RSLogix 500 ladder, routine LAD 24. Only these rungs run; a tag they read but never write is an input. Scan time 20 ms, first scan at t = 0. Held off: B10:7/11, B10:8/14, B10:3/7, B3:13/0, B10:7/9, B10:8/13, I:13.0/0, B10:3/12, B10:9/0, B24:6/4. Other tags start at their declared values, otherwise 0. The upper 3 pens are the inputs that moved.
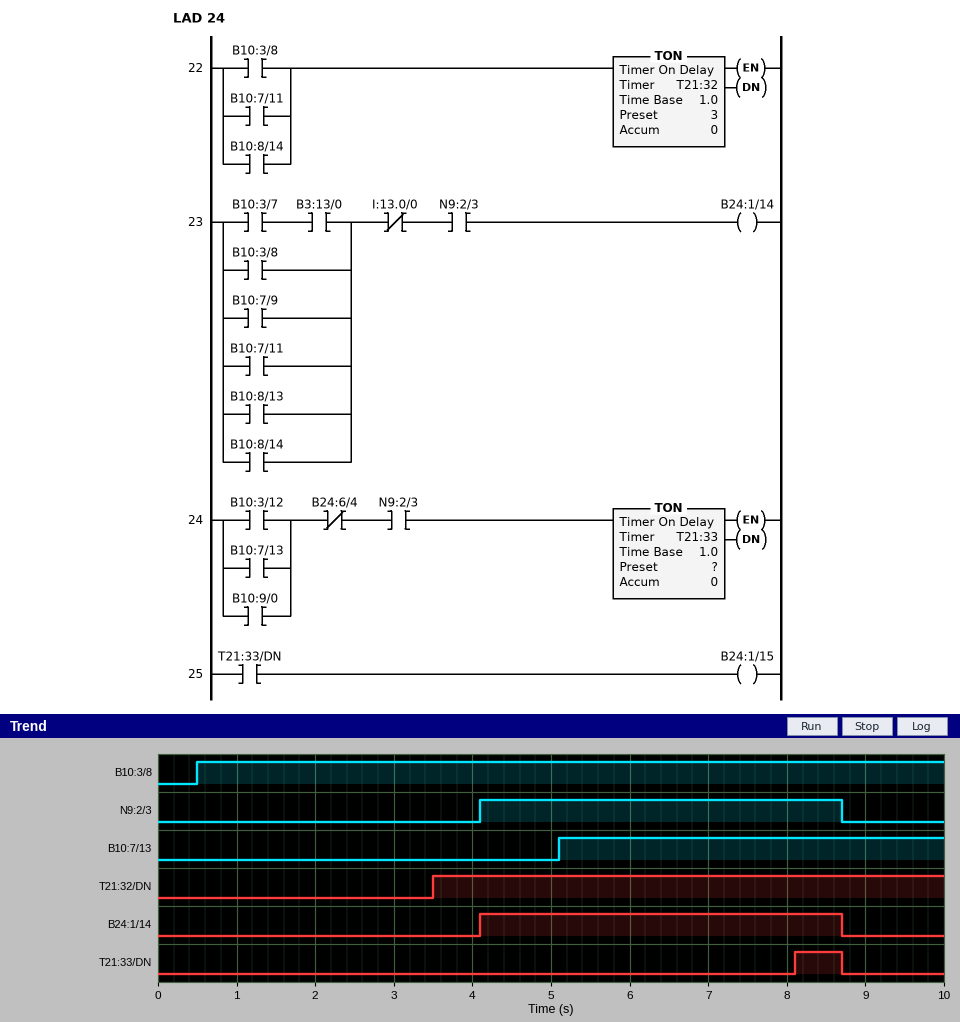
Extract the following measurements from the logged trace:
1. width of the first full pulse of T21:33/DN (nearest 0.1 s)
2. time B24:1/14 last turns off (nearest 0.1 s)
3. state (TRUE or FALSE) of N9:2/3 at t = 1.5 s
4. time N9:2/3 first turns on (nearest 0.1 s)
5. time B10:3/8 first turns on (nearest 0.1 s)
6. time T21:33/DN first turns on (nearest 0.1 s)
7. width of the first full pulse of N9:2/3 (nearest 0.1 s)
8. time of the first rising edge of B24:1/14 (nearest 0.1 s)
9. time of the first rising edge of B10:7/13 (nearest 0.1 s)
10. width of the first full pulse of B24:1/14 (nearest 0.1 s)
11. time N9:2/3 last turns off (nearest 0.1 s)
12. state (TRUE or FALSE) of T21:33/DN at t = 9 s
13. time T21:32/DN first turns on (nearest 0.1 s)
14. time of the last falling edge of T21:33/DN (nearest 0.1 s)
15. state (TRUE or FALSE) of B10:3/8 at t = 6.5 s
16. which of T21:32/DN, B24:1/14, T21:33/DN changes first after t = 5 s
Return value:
0.6 s
8.7 s
FALSE
4.1 s
0.5 s
8.1 s
4.6 s
4.1 s
5.1 s
4.6 s
8.7 s
FALSE
3.5 s
8.7 s
TRUE
T21:33/DN
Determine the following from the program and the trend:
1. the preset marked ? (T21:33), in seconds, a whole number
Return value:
3 s
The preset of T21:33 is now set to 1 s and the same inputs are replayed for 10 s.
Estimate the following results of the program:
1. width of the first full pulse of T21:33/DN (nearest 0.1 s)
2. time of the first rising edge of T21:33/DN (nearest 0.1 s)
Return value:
2.6 s
6.1 s
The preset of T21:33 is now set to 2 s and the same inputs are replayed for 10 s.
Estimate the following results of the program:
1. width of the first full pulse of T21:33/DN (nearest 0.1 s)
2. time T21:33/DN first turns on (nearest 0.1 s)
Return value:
1.6 s
7.1 s
